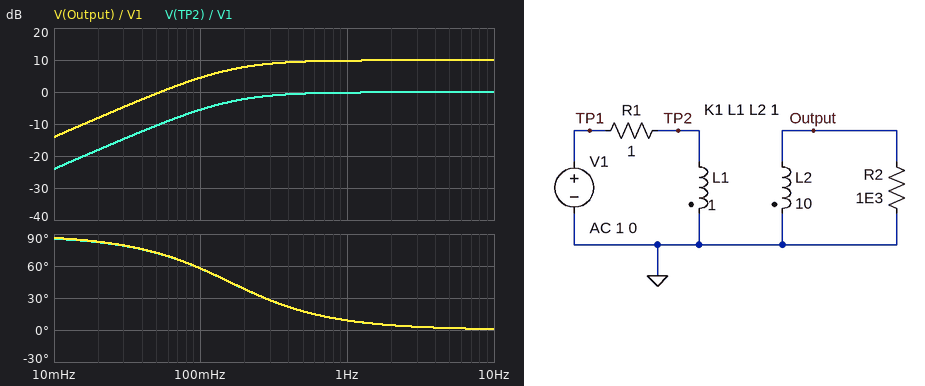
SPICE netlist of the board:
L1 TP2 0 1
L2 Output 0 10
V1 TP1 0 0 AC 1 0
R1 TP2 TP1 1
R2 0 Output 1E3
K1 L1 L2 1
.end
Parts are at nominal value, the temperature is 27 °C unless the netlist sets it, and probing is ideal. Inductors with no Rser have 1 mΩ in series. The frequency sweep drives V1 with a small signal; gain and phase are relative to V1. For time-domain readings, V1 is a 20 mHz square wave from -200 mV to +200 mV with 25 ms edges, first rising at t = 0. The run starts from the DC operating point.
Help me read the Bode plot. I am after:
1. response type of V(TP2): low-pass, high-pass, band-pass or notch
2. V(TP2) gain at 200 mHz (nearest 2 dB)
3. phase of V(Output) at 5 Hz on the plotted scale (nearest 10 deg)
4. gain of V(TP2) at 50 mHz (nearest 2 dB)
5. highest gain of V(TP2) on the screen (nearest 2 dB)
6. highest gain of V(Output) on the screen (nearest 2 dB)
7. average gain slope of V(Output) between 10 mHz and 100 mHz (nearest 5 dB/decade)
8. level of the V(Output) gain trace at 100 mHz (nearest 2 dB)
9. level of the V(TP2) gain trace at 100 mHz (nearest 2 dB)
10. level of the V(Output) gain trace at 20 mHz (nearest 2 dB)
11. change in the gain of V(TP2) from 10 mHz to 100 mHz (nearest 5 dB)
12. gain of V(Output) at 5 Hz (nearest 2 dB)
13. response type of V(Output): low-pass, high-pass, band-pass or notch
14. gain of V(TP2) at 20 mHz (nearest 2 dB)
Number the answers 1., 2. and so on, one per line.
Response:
1. high-pass
2. -2 dB
3. 0 deg
4. -10 dB
5. 0 dB
6. 10 dB
7. 20 dB/decade
8. 4 dB
9. -6 dB
10. -8 dB
11. 20 dB
12. 10 dB
13. high-pass
14. -18 dB
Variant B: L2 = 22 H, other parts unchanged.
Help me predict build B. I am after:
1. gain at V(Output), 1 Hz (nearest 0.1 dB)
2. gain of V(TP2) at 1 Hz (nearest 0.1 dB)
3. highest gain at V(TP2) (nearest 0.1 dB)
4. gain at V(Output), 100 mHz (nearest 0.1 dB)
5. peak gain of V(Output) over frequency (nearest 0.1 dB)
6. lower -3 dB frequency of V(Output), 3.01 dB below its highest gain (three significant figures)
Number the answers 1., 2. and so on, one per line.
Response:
1. 13.1 dB
2. -0.3 dB
3. -0.2 dB
4. 7.9 dB
5. 13.2 dB
6. 156 mHz
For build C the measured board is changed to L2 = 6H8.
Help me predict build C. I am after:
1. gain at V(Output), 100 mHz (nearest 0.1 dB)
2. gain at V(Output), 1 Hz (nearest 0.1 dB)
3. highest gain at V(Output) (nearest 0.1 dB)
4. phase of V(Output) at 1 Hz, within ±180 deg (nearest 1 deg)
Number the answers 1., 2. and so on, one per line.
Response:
1. 2.8 dB
2. 8.2 dB
3. 8.3 dB
4. 9 deg
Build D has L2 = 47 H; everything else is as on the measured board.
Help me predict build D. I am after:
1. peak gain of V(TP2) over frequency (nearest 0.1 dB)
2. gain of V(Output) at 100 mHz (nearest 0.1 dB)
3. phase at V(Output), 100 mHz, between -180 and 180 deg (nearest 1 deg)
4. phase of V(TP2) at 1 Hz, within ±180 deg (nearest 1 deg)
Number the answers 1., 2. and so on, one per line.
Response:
1. -0.4 dB
2. 11.1 dB
3. 57 deg
4. 9 deg
